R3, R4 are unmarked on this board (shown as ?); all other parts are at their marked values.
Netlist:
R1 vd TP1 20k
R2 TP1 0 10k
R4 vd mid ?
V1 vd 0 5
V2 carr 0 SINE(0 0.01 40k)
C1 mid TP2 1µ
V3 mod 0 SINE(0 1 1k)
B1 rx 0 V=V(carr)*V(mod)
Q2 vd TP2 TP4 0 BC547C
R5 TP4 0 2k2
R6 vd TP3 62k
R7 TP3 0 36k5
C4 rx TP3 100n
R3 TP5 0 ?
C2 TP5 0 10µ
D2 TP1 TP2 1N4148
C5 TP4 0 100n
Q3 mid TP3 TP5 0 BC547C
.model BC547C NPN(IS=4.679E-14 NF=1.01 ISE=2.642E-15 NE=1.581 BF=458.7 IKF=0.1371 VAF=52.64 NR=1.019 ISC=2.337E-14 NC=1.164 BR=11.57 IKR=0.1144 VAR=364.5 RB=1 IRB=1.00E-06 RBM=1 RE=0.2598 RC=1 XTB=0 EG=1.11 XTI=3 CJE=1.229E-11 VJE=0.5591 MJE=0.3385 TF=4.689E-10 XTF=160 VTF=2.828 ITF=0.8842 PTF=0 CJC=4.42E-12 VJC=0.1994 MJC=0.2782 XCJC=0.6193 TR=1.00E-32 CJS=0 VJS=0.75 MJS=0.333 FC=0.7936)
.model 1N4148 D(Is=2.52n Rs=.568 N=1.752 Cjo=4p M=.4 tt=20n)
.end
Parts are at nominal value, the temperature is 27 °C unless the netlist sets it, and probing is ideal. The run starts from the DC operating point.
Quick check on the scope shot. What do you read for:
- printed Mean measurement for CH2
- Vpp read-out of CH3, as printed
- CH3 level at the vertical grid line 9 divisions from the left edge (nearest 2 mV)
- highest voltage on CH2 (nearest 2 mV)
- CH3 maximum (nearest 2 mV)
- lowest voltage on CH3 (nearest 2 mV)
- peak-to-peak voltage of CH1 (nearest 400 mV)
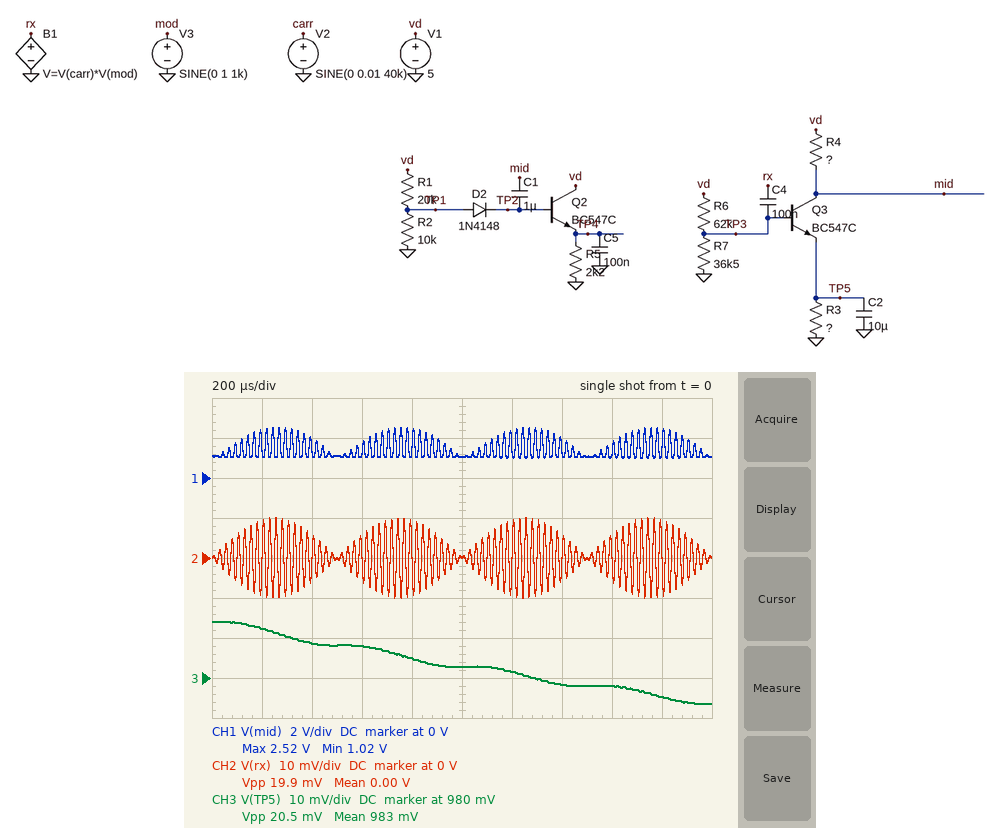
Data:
0.00 V
20.5 mV
976 mV
10 mV
994 mV
974 mV
1.6 V
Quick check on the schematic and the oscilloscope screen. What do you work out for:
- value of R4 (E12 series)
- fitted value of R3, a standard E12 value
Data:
2.7 kΩ
680 Ω
